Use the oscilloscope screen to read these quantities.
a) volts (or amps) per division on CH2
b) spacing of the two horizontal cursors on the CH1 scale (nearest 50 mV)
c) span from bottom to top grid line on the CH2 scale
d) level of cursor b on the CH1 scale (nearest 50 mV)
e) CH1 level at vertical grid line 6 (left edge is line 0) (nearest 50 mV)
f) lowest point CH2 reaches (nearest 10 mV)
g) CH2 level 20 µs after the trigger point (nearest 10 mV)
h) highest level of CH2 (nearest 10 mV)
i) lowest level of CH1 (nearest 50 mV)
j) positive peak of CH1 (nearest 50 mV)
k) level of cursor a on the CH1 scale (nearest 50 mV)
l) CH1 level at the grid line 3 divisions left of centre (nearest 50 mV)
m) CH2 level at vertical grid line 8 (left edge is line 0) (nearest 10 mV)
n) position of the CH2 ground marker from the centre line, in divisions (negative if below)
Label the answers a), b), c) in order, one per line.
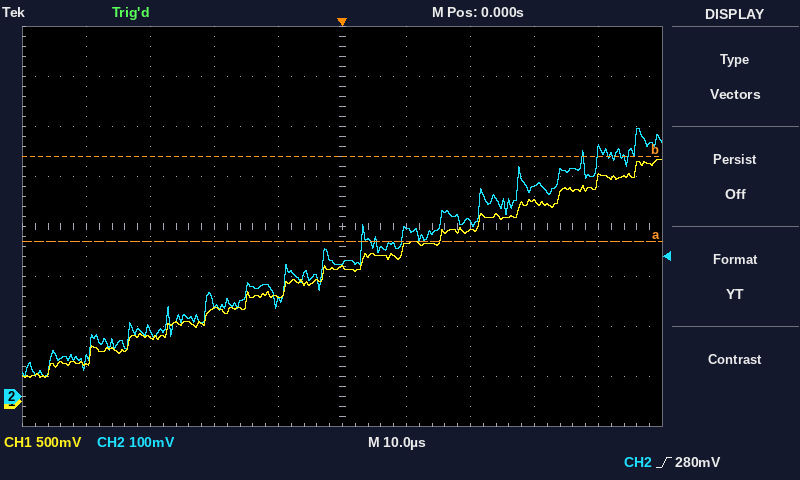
a) 100 mV
b) 850 mV
c) 800 mV
d) 2.45 V
e) 1.55 V
f) 40 mV
g) 350 mV
h) 540 mV
i) 250 mV
j) 2.40 V
k) 1.60 V
l) 650 mV
m) 420 mV
n) -3.4 div
